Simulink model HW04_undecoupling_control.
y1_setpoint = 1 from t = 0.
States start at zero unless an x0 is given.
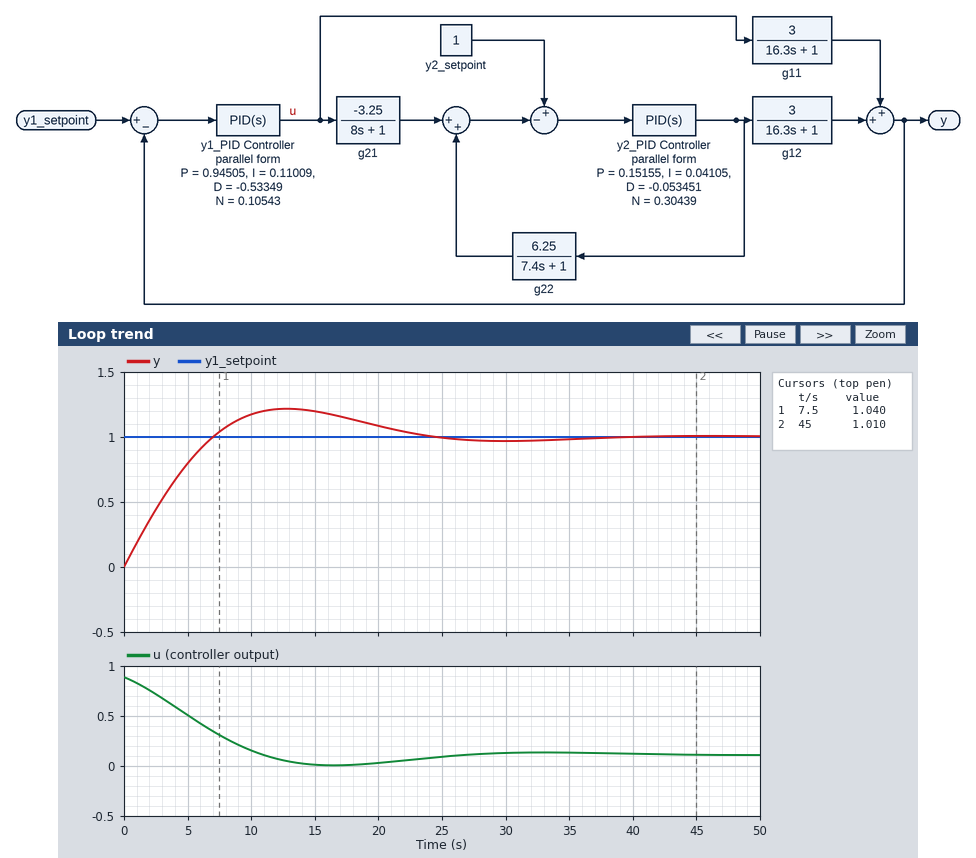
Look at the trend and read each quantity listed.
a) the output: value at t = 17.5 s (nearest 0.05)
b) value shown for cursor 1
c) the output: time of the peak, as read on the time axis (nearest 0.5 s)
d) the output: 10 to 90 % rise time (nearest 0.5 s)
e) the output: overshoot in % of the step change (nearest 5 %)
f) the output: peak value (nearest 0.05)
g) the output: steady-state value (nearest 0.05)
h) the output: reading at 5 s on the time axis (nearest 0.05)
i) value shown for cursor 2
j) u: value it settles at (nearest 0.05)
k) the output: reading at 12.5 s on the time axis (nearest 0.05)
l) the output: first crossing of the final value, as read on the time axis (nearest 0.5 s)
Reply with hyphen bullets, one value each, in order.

- 1.15
- 1.040
- 13.0 s
- 5.5 s
- 20 %
- 1.20
- 1.00
- 0.80
- 1.010
- 0.10
- 1.20
- 7.0 s
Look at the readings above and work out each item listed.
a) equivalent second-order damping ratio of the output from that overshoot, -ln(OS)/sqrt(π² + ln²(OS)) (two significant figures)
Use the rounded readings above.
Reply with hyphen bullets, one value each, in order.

- 0.46
